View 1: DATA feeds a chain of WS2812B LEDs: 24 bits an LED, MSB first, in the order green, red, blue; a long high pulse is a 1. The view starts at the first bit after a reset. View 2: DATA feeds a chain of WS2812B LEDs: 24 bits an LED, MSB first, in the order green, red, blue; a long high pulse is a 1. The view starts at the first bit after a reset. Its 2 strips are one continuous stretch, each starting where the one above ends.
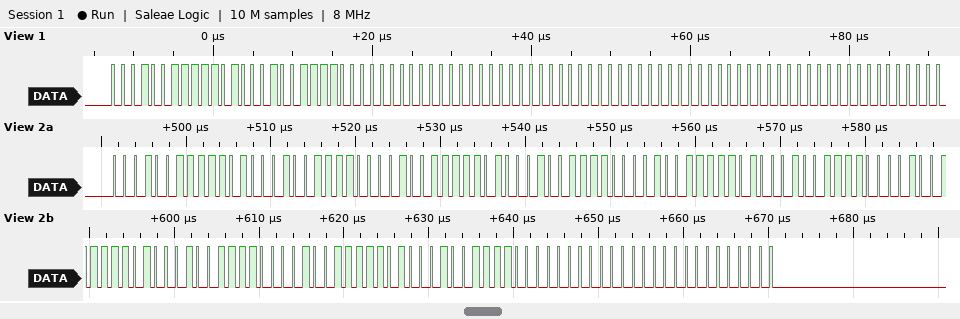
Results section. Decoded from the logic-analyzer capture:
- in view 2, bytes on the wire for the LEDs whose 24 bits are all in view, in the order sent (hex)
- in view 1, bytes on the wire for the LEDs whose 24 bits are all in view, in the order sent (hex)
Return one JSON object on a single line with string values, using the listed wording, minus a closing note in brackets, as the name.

{"in view 2, bytes on the wire for the LEDs whose 24 bits are all in view, in the order sent": "13 E8 9E 13 E8 9E 13 E8 9E 13 E8 9E 13 E8 9E 00 00 00", "in view 1, bytes on the wire for the LEDs whose 24 bits are all in view, in the order sent": "13 E8 9E 00 00 00 00 00 00"}
